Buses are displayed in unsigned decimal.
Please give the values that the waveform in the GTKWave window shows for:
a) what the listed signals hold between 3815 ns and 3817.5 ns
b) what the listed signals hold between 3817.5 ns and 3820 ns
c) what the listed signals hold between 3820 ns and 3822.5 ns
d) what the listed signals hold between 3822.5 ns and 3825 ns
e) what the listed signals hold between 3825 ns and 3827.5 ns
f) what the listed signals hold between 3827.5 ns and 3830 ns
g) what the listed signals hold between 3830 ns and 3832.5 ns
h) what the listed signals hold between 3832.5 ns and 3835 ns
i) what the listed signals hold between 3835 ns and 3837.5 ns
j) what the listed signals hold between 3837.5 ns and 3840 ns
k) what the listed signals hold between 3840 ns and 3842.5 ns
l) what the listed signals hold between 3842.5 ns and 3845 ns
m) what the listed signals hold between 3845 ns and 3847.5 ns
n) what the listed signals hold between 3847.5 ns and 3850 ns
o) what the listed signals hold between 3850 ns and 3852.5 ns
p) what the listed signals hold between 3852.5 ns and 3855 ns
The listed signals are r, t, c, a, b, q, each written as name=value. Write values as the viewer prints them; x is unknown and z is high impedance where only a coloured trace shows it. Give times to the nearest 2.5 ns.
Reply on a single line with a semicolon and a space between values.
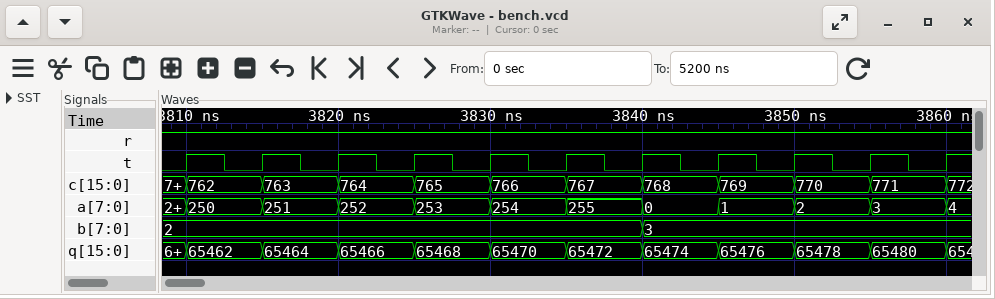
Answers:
r=1, t=1, c=763, a=251, b=2, q=65464; r=1, t=0, c=763, a=251, b=2, q=65464; r=1, t=1, c=764, a=252, b=2, q=65466; r=1, t=0, c=764, a=252, b=2, q=65466; r=1, t=1, c=765, a=253, b=2, q=65468; r=1, t=0, c=765, a=253, b=2, q=65468; r=1, t=1, c=766, a=254, b=2, q=65470; r=1, t=0, c=766, a=254, b=2, q=65470; r=1, t=1, c=767, a=255, b=2, q=65472; r=1, t=0, c=767, a=255, b=2, q=65472; r=1, t=1, c=768, a=0, b=3, q=65474; r=1, t=0, c=768, a=0, b=3, q=65474; r=1, t=1, c=769, a=1, b=3, q=65476; r=1, t=0, c=769, a=1, b=3, q=65476; r=1, t=1, c=770, a=2, b=3, q=65478; r=1, t=0, c=770, a=2, b=3, q=65478
